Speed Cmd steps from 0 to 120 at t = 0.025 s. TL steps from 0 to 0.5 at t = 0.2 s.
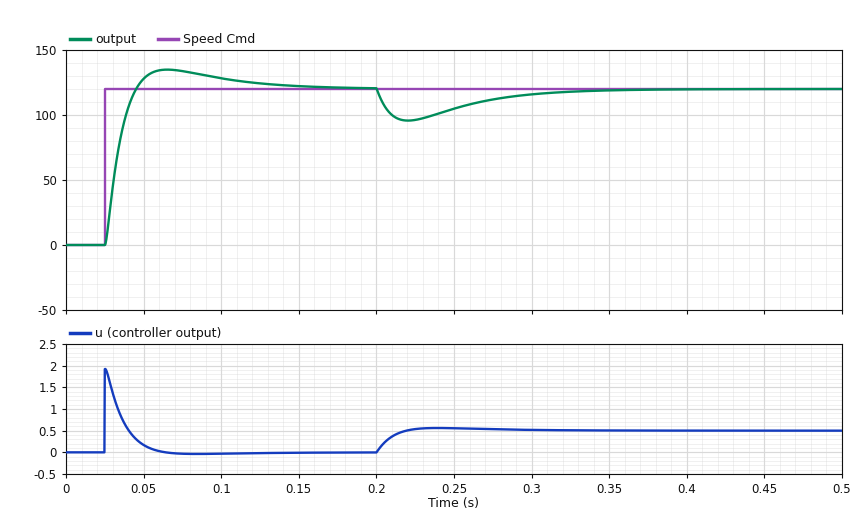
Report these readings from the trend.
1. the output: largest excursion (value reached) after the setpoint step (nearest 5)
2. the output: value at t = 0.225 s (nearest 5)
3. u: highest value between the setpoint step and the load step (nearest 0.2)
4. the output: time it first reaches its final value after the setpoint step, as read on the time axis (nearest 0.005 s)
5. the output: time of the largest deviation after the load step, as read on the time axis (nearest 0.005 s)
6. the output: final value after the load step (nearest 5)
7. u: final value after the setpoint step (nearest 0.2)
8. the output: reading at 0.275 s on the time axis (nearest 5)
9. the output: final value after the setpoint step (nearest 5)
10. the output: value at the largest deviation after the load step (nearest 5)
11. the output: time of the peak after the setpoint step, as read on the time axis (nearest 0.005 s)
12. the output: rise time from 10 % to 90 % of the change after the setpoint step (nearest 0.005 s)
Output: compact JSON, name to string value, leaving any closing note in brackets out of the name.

{"the output: largest excursion (value reached) after the setpoint step": "135", "the output: value at t = 0.225 s": "95", "u: highest value between the setpoint step and the load step": "2.0", "the output: time it first reaches its final value after the setpoint step, as read on the time axis": "0.045 s", "the output: time of the largest deviation after the load step, as read on the time axis": "0.220 s", "the output: final value after the load step": "120", "u: final value after the setpoint step": "0.0", "the output: reading at 0.275 s on the time axis": "110", "the output: final value after the setpoint step": "120", "the output: value at the largest deviation after the load step": "95", "the output: time of the peak after the setpoint step, as read on the time axis": "0.065 s", "the output: rise time from 10 % to 90 % of the change after the setpoint step": "0.015 s"}
